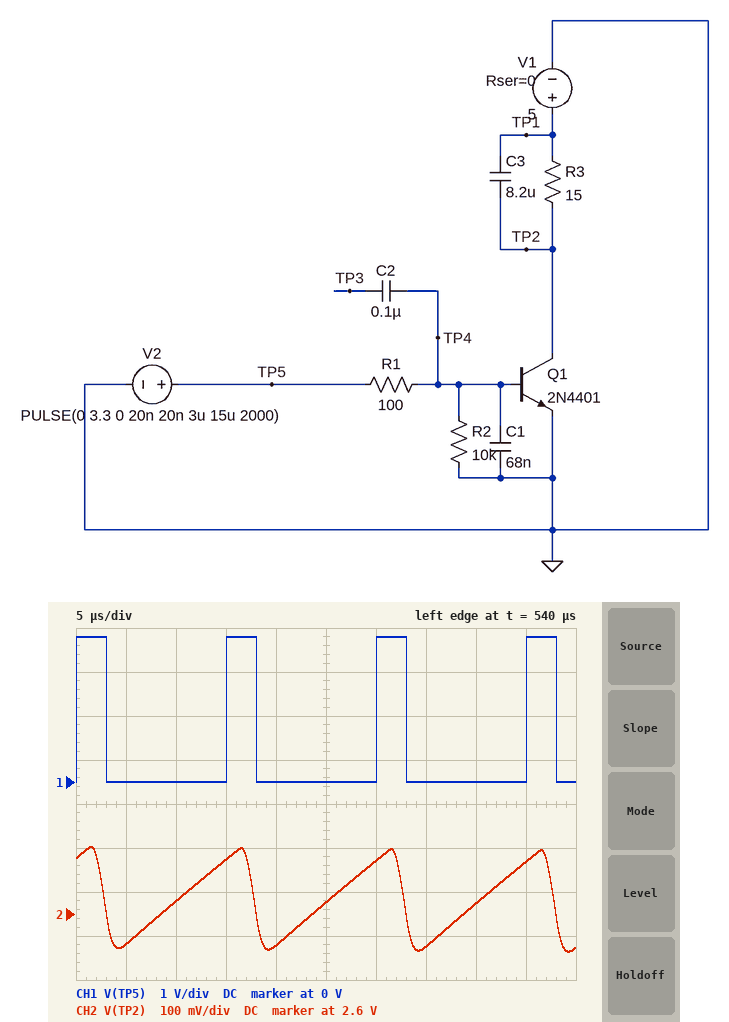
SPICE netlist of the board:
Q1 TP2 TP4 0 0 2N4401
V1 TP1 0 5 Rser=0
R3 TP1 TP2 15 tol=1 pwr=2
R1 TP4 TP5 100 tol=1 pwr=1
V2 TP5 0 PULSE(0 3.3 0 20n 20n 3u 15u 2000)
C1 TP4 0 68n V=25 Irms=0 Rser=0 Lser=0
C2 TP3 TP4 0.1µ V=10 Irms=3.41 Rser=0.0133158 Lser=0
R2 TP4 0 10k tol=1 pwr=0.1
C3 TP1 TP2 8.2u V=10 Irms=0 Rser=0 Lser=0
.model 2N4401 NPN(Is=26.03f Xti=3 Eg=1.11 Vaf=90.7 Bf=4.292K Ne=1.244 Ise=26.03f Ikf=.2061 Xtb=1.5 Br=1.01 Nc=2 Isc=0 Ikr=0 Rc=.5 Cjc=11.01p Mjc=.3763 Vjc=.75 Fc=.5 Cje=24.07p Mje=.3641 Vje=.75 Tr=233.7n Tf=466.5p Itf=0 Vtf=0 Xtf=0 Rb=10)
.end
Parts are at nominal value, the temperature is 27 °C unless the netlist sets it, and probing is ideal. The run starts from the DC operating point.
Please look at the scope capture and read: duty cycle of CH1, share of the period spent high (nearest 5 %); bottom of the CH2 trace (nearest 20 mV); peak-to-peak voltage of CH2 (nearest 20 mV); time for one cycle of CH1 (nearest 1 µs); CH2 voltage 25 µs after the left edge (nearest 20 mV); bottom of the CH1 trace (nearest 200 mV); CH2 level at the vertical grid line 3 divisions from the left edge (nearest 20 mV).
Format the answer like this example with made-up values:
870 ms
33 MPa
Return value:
20 %
2.52 V
240 mV
15 µs
2.62 V
0 V
2.72 V
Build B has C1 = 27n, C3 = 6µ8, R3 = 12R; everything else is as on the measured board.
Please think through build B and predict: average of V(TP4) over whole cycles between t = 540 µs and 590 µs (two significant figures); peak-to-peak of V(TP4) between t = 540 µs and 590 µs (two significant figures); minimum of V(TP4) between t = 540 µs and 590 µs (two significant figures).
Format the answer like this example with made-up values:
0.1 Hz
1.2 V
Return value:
350 mV
1.1 V
11 mV
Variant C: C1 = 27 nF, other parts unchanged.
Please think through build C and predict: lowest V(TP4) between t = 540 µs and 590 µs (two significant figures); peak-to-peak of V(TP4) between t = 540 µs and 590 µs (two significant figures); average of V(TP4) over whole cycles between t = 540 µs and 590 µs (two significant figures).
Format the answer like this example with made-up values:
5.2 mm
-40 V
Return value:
11 mV
1.1 V
350 mV
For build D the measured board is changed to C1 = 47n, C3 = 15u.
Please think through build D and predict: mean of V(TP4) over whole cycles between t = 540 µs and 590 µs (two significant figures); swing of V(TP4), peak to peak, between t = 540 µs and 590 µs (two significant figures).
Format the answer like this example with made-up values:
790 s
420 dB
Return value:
430 mV
1.0 V
